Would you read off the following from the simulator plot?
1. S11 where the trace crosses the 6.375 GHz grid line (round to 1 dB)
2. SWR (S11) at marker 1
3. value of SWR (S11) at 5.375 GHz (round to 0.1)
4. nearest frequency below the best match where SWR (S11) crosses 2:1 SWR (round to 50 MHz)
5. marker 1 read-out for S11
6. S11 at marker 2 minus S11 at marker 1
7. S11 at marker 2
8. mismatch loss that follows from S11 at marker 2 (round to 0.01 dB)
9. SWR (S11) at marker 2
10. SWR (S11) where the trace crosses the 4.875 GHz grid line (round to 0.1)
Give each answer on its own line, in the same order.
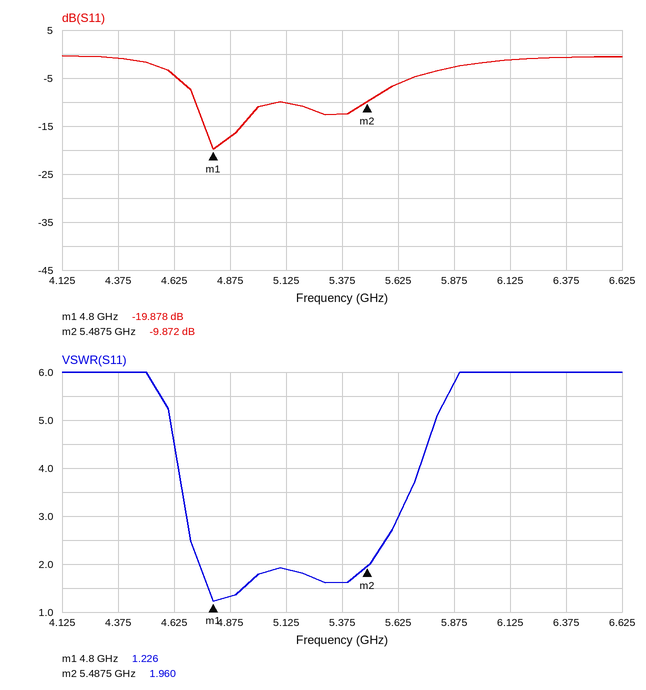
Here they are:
-1 dB
1.226
1.6
4.75 GHz
-19.878 dB
10.006 dB
-9.872 dB
0.47 dB
1.960
1.3
